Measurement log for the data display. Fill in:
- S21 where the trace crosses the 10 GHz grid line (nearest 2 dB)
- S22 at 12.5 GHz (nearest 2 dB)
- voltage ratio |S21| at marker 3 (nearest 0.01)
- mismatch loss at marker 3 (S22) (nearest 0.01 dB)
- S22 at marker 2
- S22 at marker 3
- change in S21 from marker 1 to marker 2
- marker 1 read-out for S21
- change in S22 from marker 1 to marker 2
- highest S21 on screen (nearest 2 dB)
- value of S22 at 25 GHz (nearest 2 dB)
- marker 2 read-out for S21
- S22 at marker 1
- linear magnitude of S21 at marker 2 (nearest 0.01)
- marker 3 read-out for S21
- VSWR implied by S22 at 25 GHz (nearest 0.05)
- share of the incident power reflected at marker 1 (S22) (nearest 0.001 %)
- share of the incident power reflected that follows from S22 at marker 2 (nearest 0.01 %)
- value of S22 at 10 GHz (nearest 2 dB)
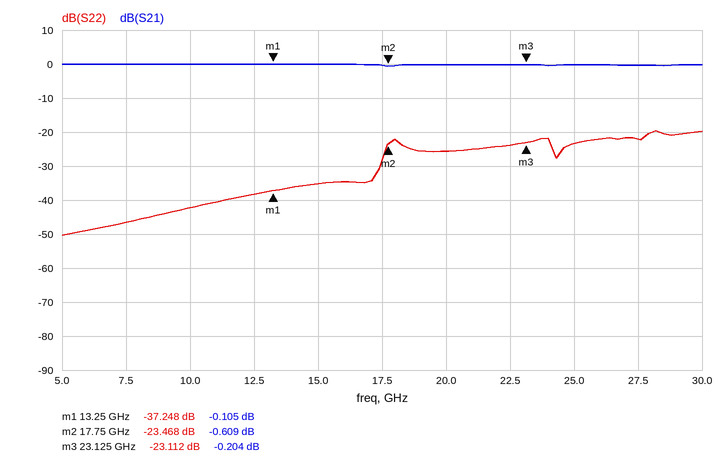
0 dB
-38 dB
0.98
0.02 dB
-23.468 dB
-23.112 dB
-0.504 dB
-0.105 dB
13.780 dB
0 dB
-24 dB
-0.609 dB
-37.248 dB
0.93
-0.204 dB
1.15
0.019 %
0.45 %
-42 dB
